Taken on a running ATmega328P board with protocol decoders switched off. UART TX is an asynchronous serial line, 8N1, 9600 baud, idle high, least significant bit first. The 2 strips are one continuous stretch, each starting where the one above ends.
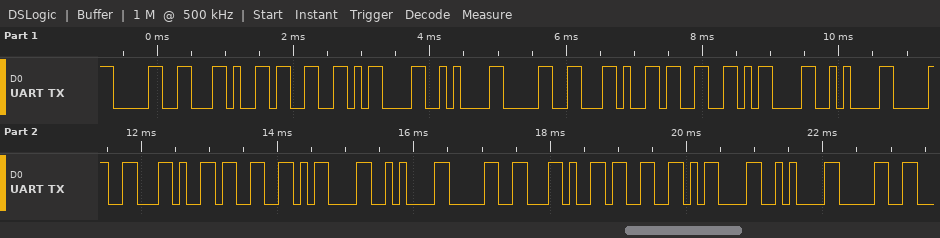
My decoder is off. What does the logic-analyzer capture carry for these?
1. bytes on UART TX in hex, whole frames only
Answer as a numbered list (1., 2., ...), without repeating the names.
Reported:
1. 30 2C 33 0D 0A 30 2C 33 0D 0A 30 2C 33 0D 0A 30 2C 33 0D 0A 30
